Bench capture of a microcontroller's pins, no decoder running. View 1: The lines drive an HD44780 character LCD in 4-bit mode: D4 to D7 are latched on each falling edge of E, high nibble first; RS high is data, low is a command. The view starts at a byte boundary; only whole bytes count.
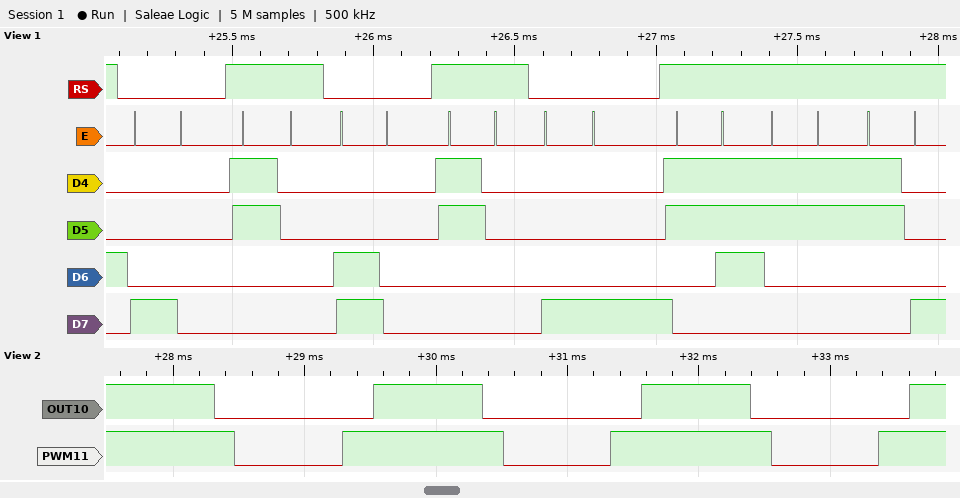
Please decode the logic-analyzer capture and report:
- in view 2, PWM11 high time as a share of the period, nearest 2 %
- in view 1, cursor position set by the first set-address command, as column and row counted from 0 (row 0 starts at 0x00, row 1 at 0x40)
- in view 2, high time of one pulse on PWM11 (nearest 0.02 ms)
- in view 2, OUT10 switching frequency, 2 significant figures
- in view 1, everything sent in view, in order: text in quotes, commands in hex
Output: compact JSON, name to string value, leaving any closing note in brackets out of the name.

{"in view 2, PWM11 high time as a share of the period, nearest 2 %": "60 %", "in view 1, cursor position set by the first set-address command, as column and row counted from 0": "column 0, row 0", "in view 2, high time of one pulse on PWM11": "1.22 ms", "in view 2, OUT10 switching frequency, 2 significant figures": "490 Hz", "in view 1, everything sent in view, in order: text in quotes, commands in hex": "0x80 \"0\" 0xC0 \"0\" 0x88 \"738\""}
